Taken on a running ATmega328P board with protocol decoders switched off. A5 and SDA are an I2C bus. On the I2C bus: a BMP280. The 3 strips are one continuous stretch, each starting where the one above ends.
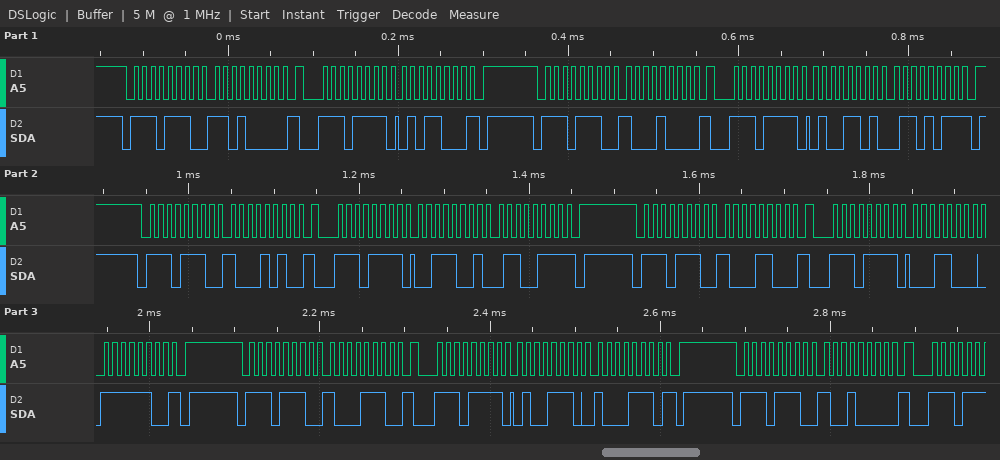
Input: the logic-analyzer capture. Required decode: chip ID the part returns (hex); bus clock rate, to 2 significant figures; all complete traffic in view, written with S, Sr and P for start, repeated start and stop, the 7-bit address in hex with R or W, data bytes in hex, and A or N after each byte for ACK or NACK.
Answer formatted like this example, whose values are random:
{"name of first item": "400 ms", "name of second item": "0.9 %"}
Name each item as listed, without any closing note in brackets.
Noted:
{"chip ID the part returns": "0x58", "bus clock rate, to 2 significant figures": "100 kHz", "all complete traffic in view, written with S, Sr and P for start, repeated start and stop, the 7-bit address in hex with R or W, data bytes in hex, and A or N after each byte for ACK or NACK": "S 77W A D0 A Sr 77R A 58 N P S 77W A 88 A Sr 77R A 4D A 6B N P S 77W A 8A A Sr 77R A 39 A 67 N P S 77W A 8C A Sr 77R A 18 A FC N P S 77W A 8E A Sr 77R A 4E A 8E N P S 77W A 90 A"}
